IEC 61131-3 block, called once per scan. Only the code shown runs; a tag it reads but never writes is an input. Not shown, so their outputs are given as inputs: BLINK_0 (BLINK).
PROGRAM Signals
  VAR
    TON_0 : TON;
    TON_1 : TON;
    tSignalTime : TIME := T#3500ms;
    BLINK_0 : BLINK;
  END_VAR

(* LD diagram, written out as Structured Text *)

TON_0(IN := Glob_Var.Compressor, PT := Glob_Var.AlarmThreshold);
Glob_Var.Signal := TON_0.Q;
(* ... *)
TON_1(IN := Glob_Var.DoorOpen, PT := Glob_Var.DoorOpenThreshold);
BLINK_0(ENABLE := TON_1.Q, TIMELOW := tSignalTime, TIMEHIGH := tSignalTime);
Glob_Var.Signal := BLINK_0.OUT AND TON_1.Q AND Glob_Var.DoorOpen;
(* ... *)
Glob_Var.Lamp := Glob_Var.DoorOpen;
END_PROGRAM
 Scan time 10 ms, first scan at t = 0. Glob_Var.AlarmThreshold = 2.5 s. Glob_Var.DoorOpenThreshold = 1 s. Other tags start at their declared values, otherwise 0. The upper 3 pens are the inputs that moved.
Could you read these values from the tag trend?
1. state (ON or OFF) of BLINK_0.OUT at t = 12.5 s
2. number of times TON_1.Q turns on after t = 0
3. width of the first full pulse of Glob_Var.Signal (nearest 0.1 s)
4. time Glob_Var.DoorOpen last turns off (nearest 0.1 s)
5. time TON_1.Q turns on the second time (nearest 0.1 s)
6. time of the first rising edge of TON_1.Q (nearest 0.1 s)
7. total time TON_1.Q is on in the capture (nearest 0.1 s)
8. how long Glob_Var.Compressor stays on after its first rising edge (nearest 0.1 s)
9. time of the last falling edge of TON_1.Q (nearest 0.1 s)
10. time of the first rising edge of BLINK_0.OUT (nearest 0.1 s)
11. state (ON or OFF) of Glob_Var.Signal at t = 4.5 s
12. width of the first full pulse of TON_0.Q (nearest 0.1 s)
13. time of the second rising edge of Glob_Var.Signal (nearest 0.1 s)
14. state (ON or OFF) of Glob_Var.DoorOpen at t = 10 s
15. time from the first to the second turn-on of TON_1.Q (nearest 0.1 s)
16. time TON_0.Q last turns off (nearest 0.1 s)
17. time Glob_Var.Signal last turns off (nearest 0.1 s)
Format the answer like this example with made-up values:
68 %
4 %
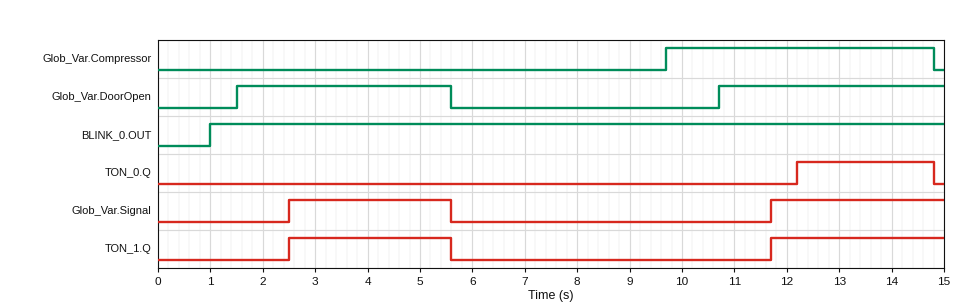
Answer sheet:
ON
2
3.1 s
5.6 s
11.7 s
2.5 s
6.4 s
5.1 s
5.6 s
1.0 s
ON
2.6 s
11.7 s
OFF
9.2 s
14.8 s
5.6 s
